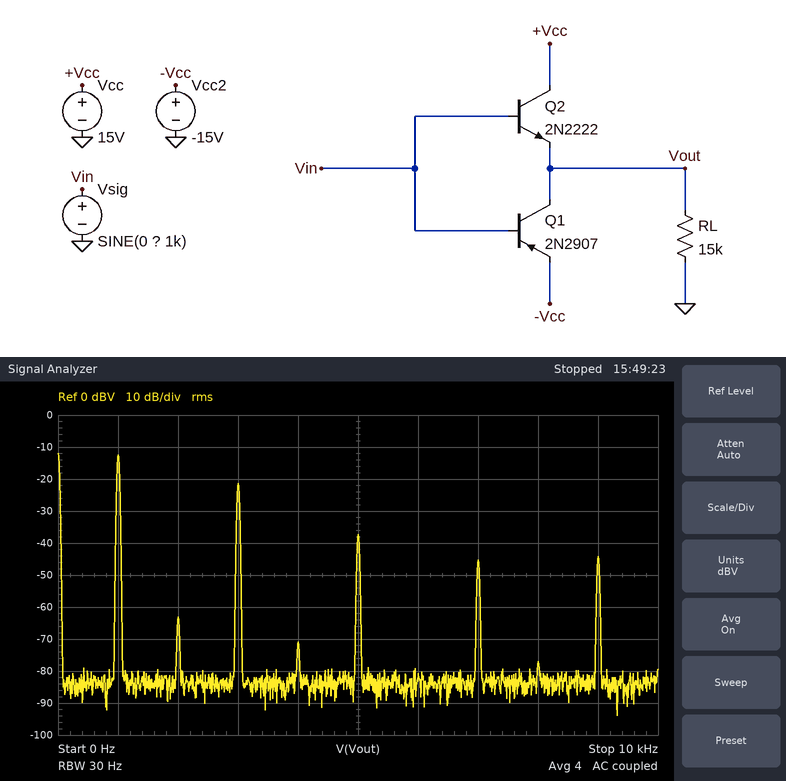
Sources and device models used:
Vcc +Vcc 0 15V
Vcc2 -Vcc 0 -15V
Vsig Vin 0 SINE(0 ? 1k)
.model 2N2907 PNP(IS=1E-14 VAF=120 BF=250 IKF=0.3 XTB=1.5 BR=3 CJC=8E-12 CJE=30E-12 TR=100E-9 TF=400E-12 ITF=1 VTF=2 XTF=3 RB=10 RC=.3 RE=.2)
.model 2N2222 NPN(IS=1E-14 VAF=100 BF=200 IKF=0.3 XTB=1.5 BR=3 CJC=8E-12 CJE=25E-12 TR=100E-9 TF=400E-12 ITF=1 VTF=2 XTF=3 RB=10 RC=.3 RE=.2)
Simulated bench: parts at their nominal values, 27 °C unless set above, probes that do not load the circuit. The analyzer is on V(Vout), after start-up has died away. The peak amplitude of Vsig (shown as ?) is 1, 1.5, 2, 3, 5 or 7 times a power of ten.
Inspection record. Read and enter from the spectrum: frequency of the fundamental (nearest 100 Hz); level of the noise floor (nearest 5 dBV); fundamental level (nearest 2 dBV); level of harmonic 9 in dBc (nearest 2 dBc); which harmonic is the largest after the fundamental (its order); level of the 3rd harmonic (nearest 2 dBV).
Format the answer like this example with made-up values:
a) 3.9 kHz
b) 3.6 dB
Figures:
a) 1.0 kHz
b) -85 dBV
c) -12 dBV
d) -32 dBc
e) 3
f) -22 dBV
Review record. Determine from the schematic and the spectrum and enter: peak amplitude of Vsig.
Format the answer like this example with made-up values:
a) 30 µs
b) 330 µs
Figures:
a) 1 V
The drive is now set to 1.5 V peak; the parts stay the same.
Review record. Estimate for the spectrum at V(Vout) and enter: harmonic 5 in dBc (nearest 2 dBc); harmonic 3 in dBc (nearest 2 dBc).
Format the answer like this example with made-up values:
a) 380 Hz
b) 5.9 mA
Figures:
a) -22 dBc
b) -14 dBc
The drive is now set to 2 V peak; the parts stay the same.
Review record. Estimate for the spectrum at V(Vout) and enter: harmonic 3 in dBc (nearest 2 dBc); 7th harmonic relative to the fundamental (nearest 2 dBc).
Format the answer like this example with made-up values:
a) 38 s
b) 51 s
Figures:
a) -16 dBc
b) -30 dBc
